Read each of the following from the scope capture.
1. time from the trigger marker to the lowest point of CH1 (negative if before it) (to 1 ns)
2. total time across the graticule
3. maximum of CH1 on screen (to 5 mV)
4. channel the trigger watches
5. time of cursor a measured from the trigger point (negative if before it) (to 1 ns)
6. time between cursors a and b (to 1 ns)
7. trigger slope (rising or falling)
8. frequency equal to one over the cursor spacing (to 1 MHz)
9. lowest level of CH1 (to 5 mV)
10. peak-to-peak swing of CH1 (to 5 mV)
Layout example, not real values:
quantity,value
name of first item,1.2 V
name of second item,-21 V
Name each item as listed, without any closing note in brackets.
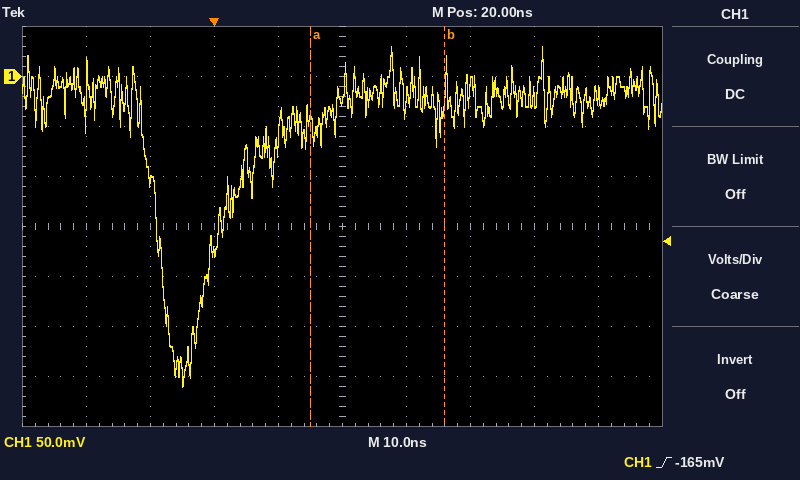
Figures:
quantity,value
time from the trigger marker to the lowest point of CH1 (negative if before it),-5 ns
total time across the graticule,100 ns
maximum of CH1 on screen,30 mV
channel the trigger watches,CH1
time of cursor a measured from the trigger point (negative if before it),+15 ns
time between cursors a and b,21 ns
trigger slope,rising
frequency equal to one over the cursor spacing,48 MHz
lowest level of CH1,-310 mV
peak-to-peak swing of CH1,340 mV
